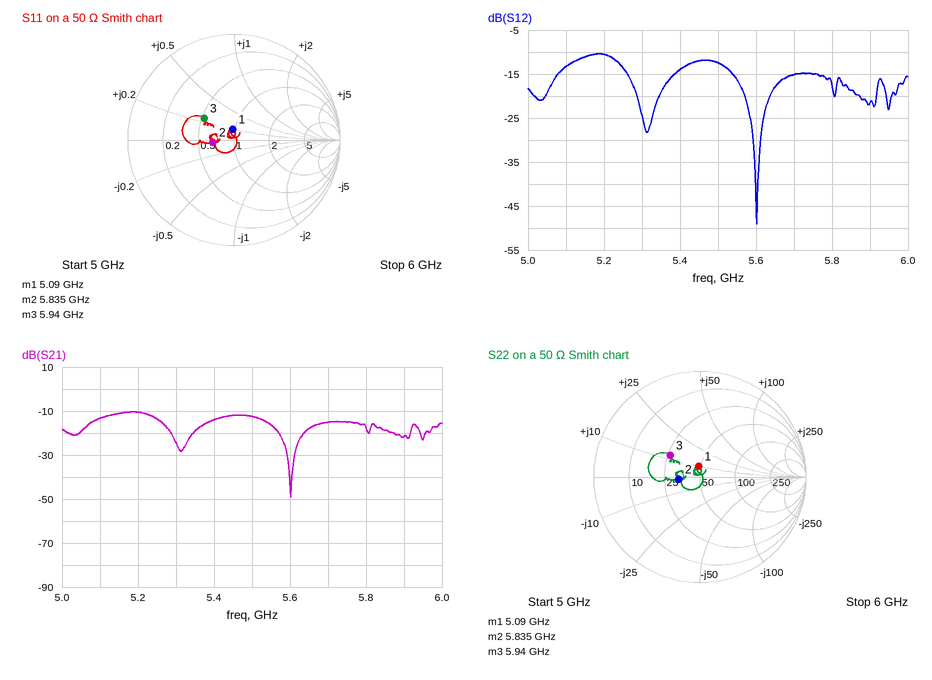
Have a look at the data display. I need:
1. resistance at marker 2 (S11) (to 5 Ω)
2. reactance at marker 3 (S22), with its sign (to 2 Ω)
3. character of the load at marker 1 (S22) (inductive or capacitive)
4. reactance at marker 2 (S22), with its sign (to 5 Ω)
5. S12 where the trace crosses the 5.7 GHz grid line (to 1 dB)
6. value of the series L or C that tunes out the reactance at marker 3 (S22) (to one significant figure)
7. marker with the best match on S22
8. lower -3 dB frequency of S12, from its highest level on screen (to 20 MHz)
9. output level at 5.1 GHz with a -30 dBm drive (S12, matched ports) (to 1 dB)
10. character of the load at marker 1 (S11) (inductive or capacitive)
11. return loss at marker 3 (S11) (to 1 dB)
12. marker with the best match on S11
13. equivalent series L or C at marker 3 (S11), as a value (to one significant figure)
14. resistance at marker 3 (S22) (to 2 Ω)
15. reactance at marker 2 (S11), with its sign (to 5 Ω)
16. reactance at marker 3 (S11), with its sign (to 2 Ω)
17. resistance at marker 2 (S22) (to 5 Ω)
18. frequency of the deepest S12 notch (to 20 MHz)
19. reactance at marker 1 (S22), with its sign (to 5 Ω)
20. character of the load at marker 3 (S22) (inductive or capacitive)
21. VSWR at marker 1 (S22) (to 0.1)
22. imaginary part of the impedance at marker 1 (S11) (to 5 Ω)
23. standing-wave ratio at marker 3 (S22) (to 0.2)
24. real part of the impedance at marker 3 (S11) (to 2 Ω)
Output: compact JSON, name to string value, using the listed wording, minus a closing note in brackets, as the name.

{"resistance at marker 2 (S11)": "35 Ω", "reactance at marker 3 (S22), with its sign": "+12 Ω", "character of the load at marker 1 (S22)": "inductive", "reactance at marker 2 (S22), with its sign": "0 Ω", "S12 where the trace crosses the 5.7 GHz grid line": "-15 dB", "value of the series L or C that tunes out the reactance at marker 3 (S22)": "2 pF", "marker with the best match on S22": "marker 1", "lower -3 dB frequency of S12, from its highest level on screen": "5.10 GHz", "output level at 5.1 GHz with a -30 dBm drive (S12, matched ports)": "-43 dBm", "character of the load at marker 1 (S11)": "inductive", "return loss at marker 3 (S11)": "9 dB", "marker with the best match on S11": "marker 1", "equivalent series L or C at marker 3 (S11), as a value": "300 pH", "resistance at marker 3 (S22)": "26 Ω", "reactance at marker 2 (S11), with its sign": "0 Ω", "reactance at marker 3 (S11), with its sign": "+12 Ω", "resistance at marker 2 (S22)": "35 Ω", "frequency of the deepest S12 notch": "5.60 GHz", "reactance at marker 1 (S22), with its sign": "+10 Ω", "character of the load at marker 3 (S22)": "inductive", "VSWR at marker 1 (S22)": "1.2", "imaginary part of the impedance at marker 1 (S11)": "+10 Ω", "standing-wave ratio at marker 3 (S22)": "2.0", "real part of the impedance at marker 3 (S11)": "26 Ω"}
